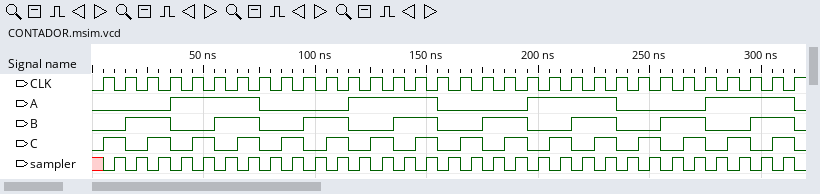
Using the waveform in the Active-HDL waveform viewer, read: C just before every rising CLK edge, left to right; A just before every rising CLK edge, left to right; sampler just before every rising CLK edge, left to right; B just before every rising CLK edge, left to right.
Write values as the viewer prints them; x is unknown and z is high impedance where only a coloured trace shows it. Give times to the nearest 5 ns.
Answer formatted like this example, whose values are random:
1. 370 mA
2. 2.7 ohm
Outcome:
1. 0 1 0 1 0 1 0 1 0 1 0 1 0 1 0 1 0 1 0 1 0 1 0 1 0 1 0 1 0 1 0 1
2. 0 0 0 0 1 1 1 1 0 0 0 0 1 1 1 1 0 0 0 0 1 1 1 1 0 0 0 0 1 1 1 1
3. x 1 1 1 1 1 1 1 1 1 1 1 1 1 1 1 1 1 1 1 1 1 1 1 1 1 1 1 1 1 1 1
4. 0 0 1 1 0 0 1 1 0 0 1 1 0 0 1 1 0 0 1 1 0 0 1 1 0 0 1 1 0 0 1 1
